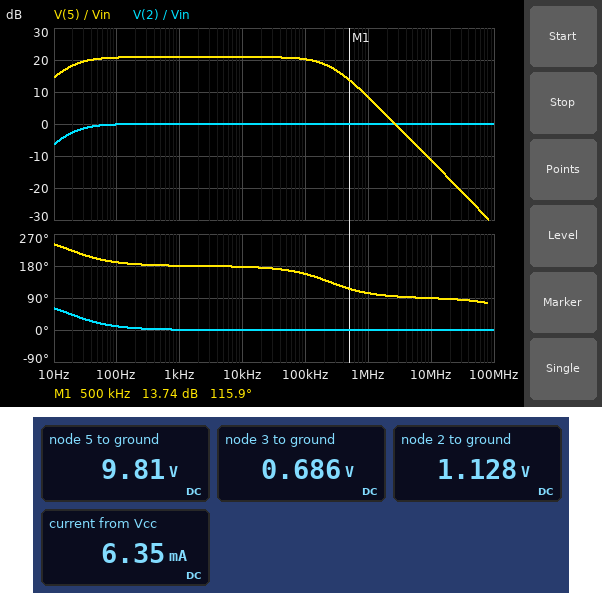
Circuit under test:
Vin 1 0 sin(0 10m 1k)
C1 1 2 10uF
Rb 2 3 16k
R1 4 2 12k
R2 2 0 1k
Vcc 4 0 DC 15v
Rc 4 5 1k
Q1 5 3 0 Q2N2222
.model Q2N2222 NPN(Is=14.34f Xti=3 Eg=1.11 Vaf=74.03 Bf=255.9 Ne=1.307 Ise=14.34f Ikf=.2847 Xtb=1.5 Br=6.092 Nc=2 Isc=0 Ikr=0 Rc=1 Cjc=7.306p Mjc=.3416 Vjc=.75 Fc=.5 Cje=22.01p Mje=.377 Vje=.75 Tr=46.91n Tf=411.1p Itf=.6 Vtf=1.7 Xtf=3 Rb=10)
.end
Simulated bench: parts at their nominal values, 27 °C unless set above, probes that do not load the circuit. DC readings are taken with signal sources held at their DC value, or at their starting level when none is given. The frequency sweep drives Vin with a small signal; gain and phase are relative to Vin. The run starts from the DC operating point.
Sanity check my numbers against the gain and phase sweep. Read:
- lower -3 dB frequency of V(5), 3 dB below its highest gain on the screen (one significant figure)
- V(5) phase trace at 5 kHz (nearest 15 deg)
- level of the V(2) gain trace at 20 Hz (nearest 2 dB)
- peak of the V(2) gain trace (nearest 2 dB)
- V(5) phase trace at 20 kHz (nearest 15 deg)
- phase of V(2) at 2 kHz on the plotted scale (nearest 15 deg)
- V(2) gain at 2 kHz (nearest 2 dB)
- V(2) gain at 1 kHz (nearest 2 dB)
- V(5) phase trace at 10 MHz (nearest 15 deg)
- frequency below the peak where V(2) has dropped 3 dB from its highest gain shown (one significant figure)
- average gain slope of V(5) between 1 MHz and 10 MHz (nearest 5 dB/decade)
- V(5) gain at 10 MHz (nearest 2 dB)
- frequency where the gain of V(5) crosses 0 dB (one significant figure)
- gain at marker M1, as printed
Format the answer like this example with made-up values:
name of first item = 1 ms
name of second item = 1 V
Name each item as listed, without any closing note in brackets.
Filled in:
lower -3 dB frequency of V(5), 3 dB below its highest gain on the screen = 20 Hz
V(5) phase trace at 5 kHz = 180 deg
level of the V(2) gain trace at 20 Hz = -2 dB
peak of the V(2) gain trace = 0 dB
V(5) phase trace at 20 kHz = 180 deg
phase of V(2) at 2 kHz on the plotted scale = 0 deg
V(2) gain at 2 kHz = 0 dB
V(2) gain at 1 kHz = 0 dB
V(5) phase trace at 10 MHz = 90 deg
frequency below the peak where V(2) has dropped 3 dB from its highest gain shown = 20 Hz
average gain slope of V(5) between 1 MHz and 10 MHz = -20 dB/decade
V(5) gain at 10 MHz = -12 dB
frequency where the gain of V(5) crosses 0 dB = 3 MHz
gain at marker M1, as printed = 13.74 dB
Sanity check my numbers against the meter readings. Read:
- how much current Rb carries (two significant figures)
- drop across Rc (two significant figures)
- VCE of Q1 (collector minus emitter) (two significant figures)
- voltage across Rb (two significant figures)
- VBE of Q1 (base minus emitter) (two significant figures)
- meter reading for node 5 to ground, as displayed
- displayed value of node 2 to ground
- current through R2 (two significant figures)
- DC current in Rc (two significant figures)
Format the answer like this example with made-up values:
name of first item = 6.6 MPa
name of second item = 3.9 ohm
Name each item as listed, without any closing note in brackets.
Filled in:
how much current Rb carries = 28 µA
drop across Rc = 5.2 V
VCE of Q1 (collector minus emitter) = 9.8 V
voltage across Rb = 440 mV
VBE of Q1 (base minus emitter) = 690 mV
meter reading for node 5 to ground, as displayed = 9.81 V
displayed value of node 2 to ground = 1.128 V
current through R2 = 1.1 mA
DC current in Rc = 5.2 mA
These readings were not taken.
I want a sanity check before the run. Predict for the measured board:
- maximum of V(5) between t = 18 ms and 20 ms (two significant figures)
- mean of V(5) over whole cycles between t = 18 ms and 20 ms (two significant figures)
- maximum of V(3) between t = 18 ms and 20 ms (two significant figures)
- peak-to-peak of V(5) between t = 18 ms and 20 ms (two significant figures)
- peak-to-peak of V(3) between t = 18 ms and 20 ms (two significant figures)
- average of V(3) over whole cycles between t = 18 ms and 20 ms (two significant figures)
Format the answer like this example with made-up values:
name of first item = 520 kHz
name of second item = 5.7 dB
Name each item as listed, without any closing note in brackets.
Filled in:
maximum of V(5) between t = 18 ms and 20 ms = 9.9 V
mean of V(5) over whole cycles between t = 18 ms and 20 ms = 9.8 V
maximum of V(3) between t = 18 ms and 20 ms = 690 mV
peak-to-peak of V(5) between t = 18 ms and 20 ms = 220 mV
peak-to-peak of V(3) between t = 18 ms and 20 ms = 1.2 mV
average of V(3) over whole cycles between t = 18 ms and 20 ms = 690 mV
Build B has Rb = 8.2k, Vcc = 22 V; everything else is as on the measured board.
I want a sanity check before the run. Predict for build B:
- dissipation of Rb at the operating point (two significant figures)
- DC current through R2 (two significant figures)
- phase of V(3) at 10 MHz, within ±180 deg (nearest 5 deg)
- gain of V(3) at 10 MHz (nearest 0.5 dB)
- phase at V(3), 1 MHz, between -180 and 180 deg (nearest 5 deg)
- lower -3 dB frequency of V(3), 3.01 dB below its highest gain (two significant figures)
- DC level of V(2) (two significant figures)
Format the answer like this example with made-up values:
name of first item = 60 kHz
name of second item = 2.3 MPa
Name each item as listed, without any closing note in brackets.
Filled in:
dissipation of Rb at the operating point = 92 µW
DC current through R2 = 1.6 mA
phase of V(3) at 10 MHz, within ±180 deg = -25 deg
gain of V(3) at 10 MHz = -56.5 dB
phase at V(3), 1 MHz, between -180 and 180 deg = -65 deg
lower -3 dB frequency of V(3), 3.01 dB below its highest gain = 19 Hz
DC level of V(2) = 1.6 V
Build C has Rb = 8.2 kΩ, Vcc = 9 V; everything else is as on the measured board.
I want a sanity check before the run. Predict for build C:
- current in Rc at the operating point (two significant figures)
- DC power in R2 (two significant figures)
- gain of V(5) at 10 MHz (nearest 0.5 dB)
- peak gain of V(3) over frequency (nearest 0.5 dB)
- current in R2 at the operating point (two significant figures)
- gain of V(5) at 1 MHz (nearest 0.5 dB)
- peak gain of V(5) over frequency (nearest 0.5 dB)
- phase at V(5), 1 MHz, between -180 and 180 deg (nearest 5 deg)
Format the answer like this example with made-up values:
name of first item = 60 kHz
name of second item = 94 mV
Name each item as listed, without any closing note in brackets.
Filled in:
current in Rc at the operating point = 900 µA
DC power in R2 = 470 µW
gain of V(5) at 10 MHz = -8.0 dB
peak gain of V(3) over frequency = -8.5 dB
current in R2 at the operating point = 690 µA
gain of V(5) at 1 MHz = 11.5 dB
peak gain of V(5) over frequency = 22.5 dB
phase at V(5), 1 MHz, between -180 and 180 deg = 105 deg
